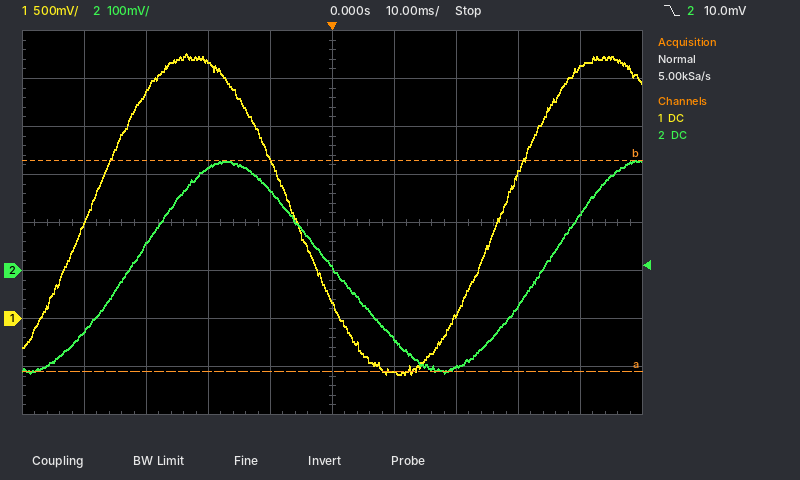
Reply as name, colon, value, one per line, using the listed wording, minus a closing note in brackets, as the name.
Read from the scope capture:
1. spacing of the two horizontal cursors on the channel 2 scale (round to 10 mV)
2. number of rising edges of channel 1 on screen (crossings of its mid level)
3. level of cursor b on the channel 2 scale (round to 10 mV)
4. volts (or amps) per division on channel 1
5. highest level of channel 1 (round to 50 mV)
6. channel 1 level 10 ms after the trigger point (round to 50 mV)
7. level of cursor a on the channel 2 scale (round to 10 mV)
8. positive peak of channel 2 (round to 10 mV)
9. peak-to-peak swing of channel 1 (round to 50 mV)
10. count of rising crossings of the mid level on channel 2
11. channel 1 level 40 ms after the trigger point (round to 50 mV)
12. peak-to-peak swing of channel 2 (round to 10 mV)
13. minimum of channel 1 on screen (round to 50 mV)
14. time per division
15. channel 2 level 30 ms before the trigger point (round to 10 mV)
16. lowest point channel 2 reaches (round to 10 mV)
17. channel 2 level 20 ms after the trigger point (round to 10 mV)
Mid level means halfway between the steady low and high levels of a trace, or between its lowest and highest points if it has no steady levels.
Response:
spacing of the two horizontal cursors on the channel 2 scale: 440 mV
number of rising edges of channel 1 on screen: 2
level of cursor b on the channel 2 scale: 230 mV
volts (or amps) per division on channel 1: 500 mV
highest level of channel 1: 2.75 V
channel 1 level 10 ms after the trigger point: -550 mV
level of cursor a on the channel 2 scale: -210 mV
positive peak of channel 2: 230 mV
peak-to-peak swing of channel 1: 3.35 V
count of rising crossings of the mid level on channel 2: 2
channel 1 level 40 ms after the trigger point: 2.60 V
peak-to-peak swing of channel 2: 440 mV
minimum of channel 1 on screen: -600 mV
time per division: 10 ms
channel 2 level 30 ms before the trigger point: 50 mV
lowest point channel 2 reaches: -210 mV
channel 2 level 20 ms after the trigger point: -200 mV
